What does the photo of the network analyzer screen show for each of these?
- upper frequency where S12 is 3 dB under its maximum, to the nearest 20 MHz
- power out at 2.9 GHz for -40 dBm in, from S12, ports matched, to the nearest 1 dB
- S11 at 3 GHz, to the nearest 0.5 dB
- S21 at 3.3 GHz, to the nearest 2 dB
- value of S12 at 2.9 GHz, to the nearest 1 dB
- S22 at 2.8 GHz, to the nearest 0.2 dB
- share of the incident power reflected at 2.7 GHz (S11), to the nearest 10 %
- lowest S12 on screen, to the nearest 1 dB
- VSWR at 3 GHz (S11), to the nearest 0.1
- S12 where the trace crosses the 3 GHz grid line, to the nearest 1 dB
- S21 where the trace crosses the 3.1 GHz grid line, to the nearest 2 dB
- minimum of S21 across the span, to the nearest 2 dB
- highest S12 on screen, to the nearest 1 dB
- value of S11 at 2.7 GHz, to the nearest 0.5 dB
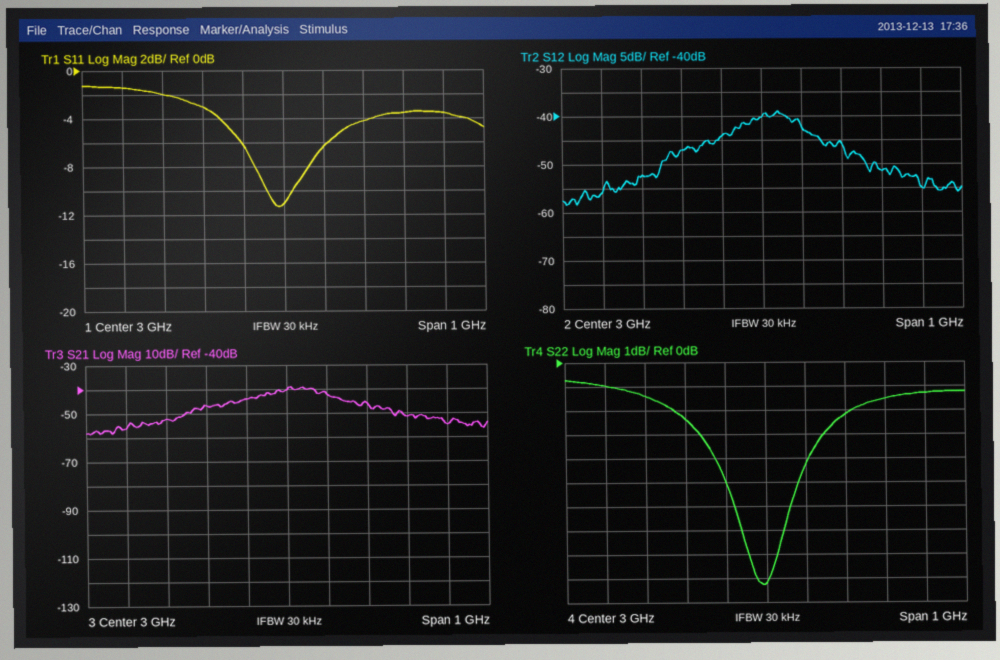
3.10 GHz
-84 dBm
-11.0 dB
-52 dB
-44 dB
-2.4 dB
60 %
-58 dB
1.8
-40 dB
-42 dB
-58 dB
-39 dB
-2.0 dB
